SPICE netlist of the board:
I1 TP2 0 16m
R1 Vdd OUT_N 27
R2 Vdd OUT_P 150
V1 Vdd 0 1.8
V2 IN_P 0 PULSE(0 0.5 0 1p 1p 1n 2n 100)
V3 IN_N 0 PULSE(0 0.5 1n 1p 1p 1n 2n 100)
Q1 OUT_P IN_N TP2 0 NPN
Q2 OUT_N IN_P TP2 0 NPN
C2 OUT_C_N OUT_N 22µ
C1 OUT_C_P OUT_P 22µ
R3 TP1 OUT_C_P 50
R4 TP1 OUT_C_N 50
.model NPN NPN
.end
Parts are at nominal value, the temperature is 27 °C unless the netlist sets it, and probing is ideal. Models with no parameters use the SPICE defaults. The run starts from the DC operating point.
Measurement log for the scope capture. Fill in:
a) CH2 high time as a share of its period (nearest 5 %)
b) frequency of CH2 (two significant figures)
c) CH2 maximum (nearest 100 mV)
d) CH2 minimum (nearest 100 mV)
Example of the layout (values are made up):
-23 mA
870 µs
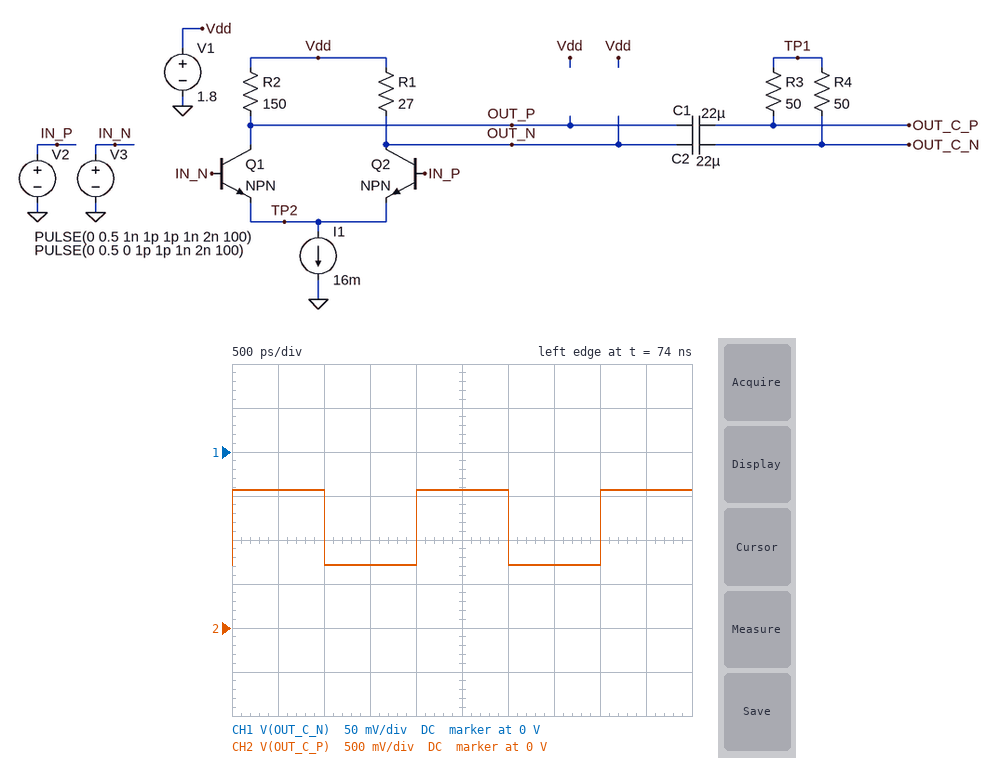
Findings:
50 %
500 MHz
1.6 V
700 mV
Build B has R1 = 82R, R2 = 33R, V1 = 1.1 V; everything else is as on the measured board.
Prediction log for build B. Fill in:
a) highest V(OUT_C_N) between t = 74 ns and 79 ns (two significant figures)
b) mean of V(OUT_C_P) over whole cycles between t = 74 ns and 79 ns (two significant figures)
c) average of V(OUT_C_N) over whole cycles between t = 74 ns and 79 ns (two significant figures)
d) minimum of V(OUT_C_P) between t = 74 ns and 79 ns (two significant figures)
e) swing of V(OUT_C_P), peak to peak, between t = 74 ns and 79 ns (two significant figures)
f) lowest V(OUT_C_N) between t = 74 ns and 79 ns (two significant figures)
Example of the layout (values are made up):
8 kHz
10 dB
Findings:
900 mV
780 mV
600 mV
660 mV
240 mV
300 mV
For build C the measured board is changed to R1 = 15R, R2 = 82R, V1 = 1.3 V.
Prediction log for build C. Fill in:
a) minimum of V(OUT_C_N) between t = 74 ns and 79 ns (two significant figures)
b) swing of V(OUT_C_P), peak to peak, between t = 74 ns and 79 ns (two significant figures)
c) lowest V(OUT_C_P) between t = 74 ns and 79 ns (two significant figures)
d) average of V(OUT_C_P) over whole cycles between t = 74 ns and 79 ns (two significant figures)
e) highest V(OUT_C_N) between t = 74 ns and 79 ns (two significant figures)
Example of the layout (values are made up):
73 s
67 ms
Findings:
1.1 V
660 mV
540 mV
870 mV
1.2 V
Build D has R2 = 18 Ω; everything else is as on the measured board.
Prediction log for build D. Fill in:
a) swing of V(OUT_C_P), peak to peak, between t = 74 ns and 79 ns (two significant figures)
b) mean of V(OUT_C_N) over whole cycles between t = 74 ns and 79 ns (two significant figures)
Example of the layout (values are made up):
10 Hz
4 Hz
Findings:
200 mV
1.6 V
